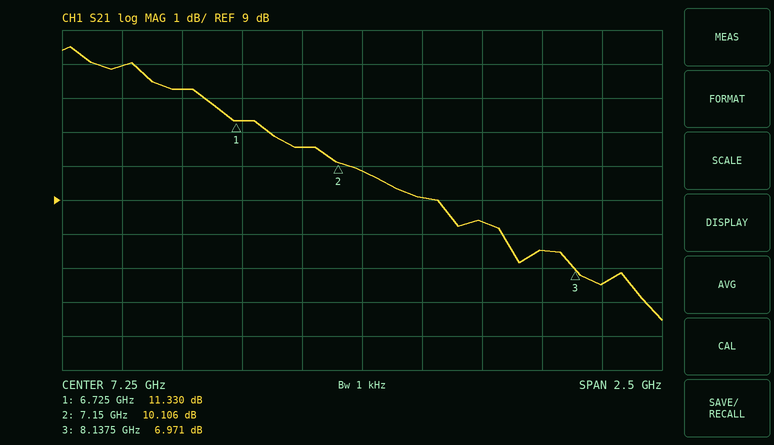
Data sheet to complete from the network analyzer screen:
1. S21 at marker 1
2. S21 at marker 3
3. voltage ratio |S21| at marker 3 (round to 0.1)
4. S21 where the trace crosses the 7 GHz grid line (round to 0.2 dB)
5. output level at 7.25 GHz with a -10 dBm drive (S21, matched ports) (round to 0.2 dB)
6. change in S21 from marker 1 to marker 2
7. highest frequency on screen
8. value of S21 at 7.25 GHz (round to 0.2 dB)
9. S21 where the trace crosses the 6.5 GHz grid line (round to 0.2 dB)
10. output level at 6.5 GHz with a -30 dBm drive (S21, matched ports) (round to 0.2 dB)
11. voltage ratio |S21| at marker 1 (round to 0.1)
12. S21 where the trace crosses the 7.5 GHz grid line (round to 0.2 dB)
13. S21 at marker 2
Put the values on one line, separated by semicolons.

11.330 dB; 6.971 dB; 2.2; 10.6 dB; -0.2 dBm; -1.224 dB; 8.5 GHz; 9.8 dB; 12.2 dB; -17.8 dBm; 3.7; 9.0 dB; 10.106 dB
